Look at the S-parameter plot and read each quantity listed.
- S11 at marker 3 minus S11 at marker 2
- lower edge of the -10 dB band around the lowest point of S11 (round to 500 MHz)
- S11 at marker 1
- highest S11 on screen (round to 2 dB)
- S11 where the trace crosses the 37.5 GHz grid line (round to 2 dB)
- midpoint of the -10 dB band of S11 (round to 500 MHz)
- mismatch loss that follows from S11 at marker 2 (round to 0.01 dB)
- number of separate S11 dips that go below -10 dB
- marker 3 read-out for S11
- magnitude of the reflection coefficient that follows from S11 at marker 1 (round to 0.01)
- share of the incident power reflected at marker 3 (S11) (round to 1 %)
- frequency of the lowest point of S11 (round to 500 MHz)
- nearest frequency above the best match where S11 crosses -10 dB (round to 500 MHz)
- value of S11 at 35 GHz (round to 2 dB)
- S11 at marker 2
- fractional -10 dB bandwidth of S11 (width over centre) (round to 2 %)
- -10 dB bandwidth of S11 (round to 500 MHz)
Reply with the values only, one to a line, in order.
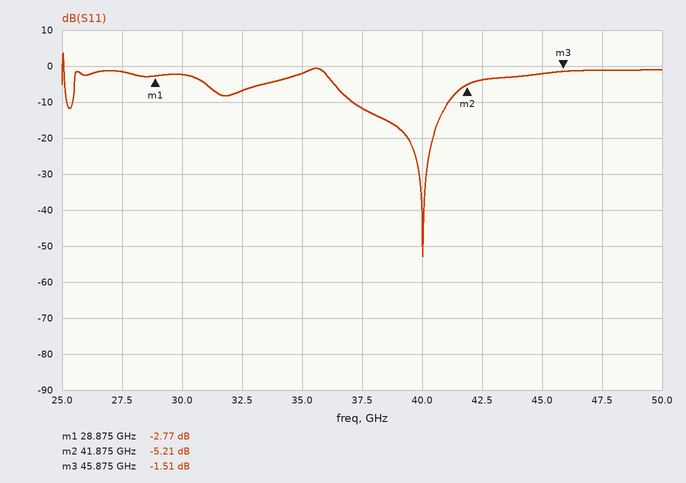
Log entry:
3.70 dB
37.0 GHz
-2.77 dB
4 dB
-12 dB
39.0 GHz
1.56 dB
2
-1.51 dB
0.73
71 %
40.0 GHz
41.0 GHz
-2 dB
-5.21 dB
10 %
4.0 GHz
